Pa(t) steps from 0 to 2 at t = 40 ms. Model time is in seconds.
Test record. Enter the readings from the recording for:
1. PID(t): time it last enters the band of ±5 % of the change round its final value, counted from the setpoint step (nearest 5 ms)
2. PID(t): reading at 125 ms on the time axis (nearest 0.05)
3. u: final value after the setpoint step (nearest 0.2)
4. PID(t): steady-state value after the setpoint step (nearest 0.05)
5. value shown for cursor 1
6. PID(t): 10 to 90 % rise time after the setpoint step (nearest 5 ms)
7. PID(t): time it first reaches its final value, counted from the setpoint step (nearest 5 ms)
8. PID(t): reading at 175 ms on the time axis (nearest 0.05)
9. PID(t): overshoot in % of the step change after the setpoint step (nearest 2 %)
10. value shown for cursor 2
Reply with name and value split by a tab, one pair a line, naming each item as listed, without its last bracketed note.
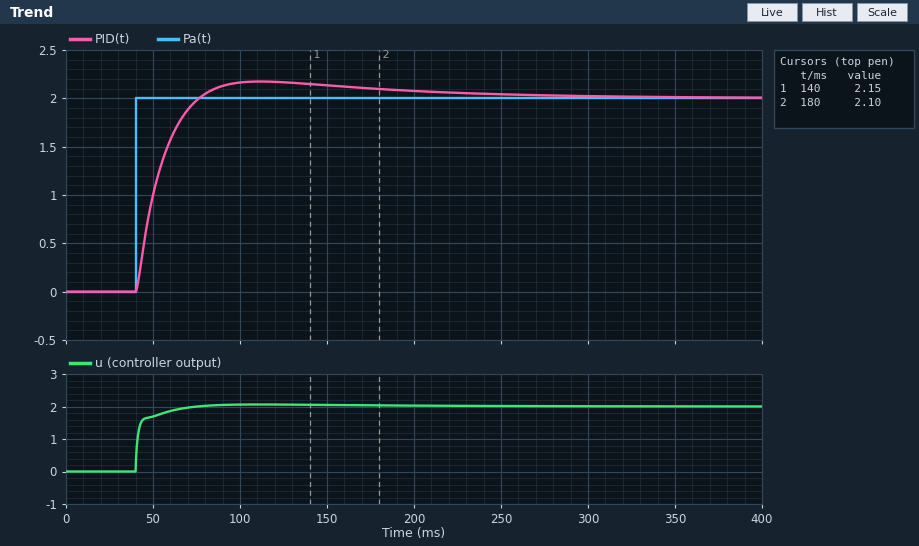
PID(t): time it last enters the band of ±5 % of the change round its final value, counted from the setpoint step	135 ms
PID(t): reading at 125 ms on the time axis	2.15
u: final value after the setpoint step	2.0
PID(t): steady-state value after the setpoint step	2.00
value shown for cursor 1	2.15
PID(t): 10 to 90 % rise time after the setpoint step	25 ms
PID(t): time it first reaches its final value, counted from the setpoint step	35 ms
PID(t): reading at 175 ms on the time axis	2.10
PID(t): overshoot in % of the step change after the setpoint step	8 %
value shown for cursor 2	2.10
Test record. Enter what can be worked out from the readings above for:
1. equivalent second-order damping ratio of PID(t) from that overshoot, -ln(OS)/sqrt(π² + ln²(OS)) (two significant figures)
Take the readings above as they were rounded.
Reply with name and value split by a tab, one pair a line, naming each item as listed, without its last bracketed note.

equivalent second-order damping ratio of PID(t) from that overshoot, -ln(OS)/sqrt(π² + ln²(OS))	0.63
